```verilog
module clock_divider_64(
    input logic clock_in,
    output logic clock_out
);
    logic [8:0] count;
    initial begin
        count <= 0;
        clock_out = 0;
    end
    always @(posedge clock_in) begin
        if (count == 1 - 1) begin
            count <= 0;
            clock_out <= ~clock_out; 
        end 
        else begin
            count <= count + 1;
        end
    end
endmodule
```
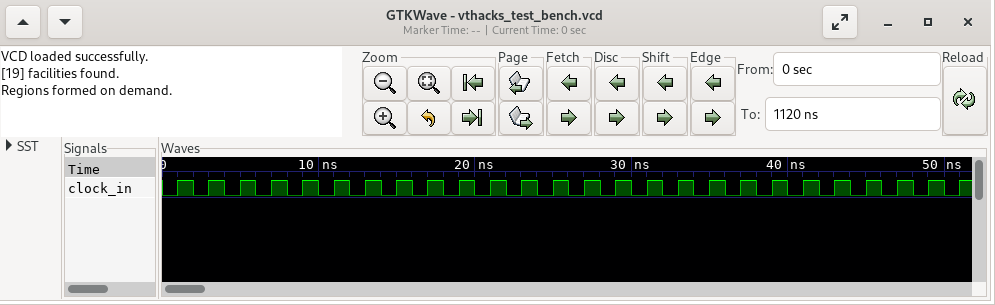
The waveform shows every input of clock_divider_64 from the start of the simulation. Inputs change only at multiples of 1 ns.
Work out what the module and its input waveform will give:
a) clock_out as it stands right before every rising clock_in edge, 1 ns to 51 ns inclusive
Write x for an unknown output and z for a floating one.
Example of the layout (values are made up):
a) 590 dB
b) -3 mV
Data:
a) 0 1 0 1 0 1 0 1 0 1 0 1 0 1 0 1 0 1 0 1 0 1 0 1 0 1
